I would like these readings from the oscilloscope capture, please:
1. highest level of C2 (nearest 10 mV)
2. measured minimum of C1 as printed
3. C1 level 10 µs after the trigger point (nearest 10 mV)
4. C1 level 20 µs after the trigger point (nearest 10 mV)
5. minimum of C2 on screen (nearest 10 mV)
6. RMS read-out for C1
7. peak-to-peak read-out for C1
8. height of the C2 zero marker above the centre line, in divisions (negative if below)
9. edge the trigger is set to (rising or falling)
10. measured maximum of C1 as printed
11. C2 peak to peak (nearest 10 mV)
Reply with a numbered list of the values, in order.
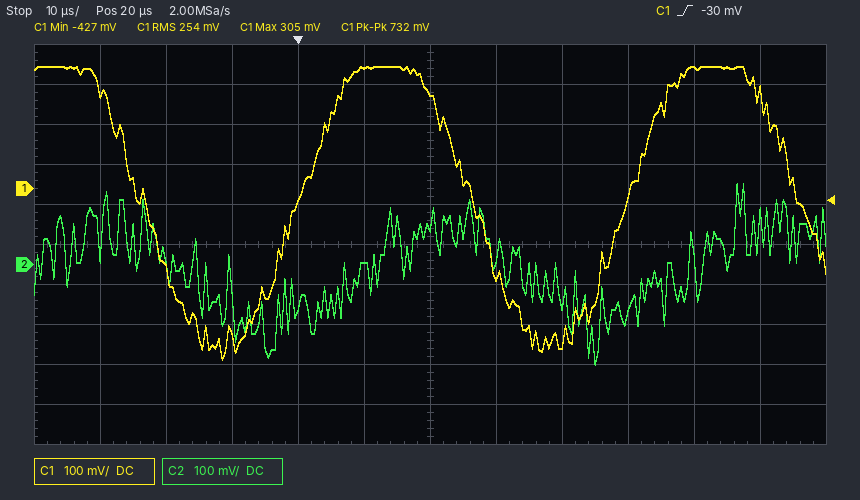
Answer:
1. 200 mV
2. -427 mV
3. 300 mV
4. 240 mV
5. -250 mV
6. 254 mV
7. 732 mV
8. -0.5 div
9. rising
10. 305 mV
11. 450 mV
